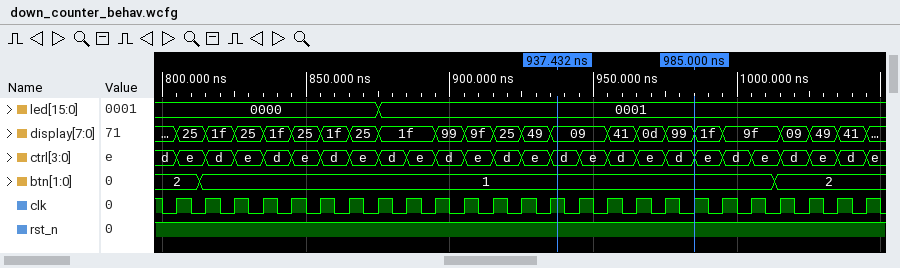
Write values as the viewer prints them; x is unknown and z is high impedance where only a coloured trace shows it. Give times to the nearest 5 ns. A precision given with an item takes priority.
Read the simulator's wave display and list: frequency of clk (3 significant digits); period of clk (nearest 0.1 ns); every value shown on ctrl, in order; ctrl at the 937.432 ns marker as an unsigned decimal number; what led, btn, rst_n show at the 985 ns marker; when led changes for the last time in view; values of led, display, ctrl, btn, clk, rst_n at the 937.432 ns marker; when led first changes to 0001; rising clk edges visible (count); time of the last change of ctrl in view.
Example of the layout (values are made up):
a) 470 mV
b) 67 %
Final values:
a) 100 MHz
b) 10 ns
c) d, e, d, e, d, e, d, e, d, e, d, e, d, e, d, e, d, e, d, e, d, e, d, e, d, e
d) 13
e) led=0001, btn=1, rst_n=1
f) 875 ns
g) led=0001, display=09, ctrl=d, btn=1, clk=1, rst_n=1
h) 875 ns
i) 25
j) 1045 ns
